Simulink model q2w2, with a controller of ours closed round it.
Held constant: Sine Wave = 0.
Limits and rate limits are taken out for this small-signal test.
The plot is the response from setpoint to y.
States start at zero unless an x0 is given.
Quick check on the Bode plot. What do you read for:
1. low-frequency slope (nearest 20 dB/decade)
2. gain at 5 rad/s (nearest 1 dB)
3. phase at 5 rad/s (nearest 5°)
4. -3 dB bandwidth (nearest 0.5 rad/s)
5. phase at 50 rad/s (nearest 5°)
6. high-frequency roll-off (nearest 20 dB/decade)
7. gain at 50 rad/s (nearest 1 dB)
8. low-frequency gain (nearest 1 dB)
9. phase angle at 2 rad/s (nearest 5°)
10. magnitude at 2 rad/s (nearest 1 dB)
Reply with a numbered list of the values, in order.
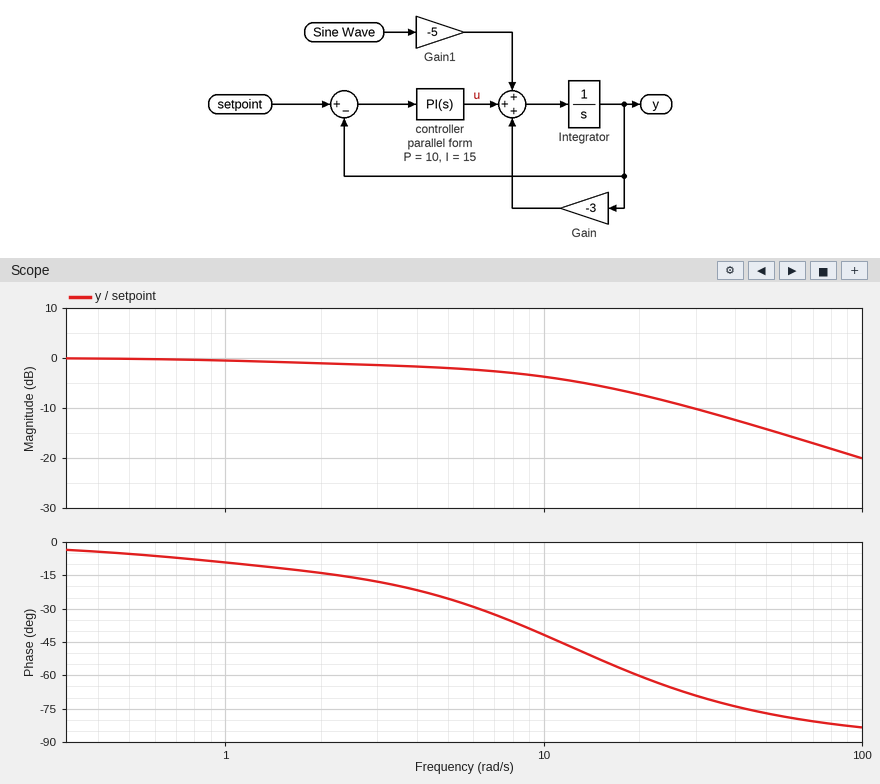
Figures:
1. 0 dB/decade
2. -2 dB
3. -25°
4. 8.5 rad/s
5. -75°
6. -20 dB/decade
7. -14 dB
8. 0 dB
9. -15°
10. -1 dB
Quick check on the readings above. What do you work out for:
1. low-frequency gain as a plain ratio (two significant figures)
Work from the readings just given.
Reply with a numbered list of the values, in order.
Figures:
1. 1.0
